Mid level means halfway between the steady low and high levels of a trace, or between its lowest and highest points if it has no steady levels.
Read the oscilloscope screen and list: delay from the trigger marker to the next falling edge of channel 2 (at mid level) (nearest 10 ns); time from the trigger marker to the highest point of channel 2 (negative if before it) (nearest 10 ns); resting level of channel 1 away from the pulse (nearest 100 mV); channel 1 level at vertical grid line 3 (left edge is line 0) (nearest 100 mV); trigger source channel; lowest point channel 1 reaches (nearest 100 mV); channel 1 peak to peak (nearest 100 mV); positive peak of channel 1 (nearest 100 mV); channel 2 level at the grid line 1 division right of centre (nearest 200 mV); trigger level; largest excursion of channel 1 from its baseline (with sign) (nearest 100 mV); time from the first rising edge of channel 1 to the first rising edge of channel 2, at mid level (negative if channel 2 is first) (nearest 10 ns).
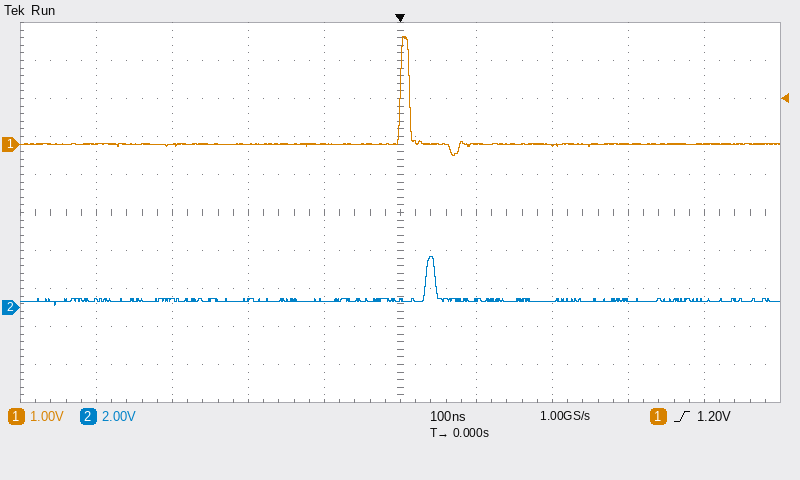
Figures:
50 ns
+40 ns
0.0 V
0.0 V
channel 1
-300 mV
3.1 V
2.8 V
400 mV
1.20 V
+2.8 V
+30 ns
